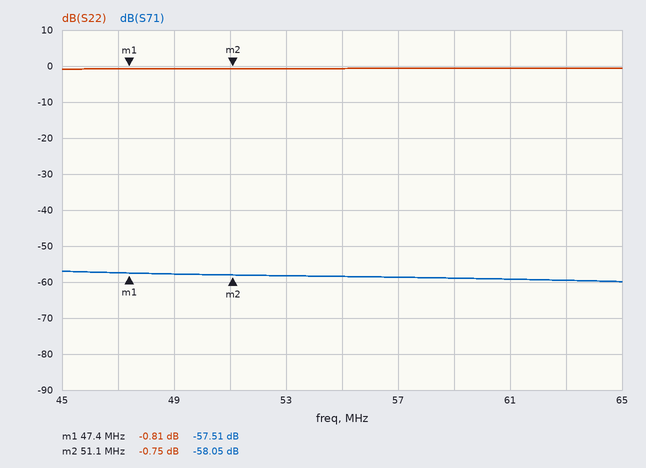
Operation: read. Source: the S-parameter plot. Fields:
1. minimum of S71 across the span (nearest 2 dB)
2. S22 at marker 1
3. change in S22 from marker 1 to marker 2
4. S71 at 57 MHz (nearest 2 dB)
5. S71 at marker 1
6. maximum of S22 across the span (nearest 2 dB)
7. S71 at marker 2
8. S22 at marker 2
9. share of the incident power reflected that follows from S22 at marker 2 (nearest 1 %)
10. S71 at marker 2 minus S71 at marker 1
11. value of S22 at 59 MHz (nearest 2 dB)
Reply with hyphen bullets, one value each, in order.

- -60 dB
- -0.81 dB
- 0.06 dB
- -58 dB
- -57.51 dB
- 0 dB
- -58.05 dB
- -0.75 dB
- 84 %
- -0.54 dB
- 0 dB
